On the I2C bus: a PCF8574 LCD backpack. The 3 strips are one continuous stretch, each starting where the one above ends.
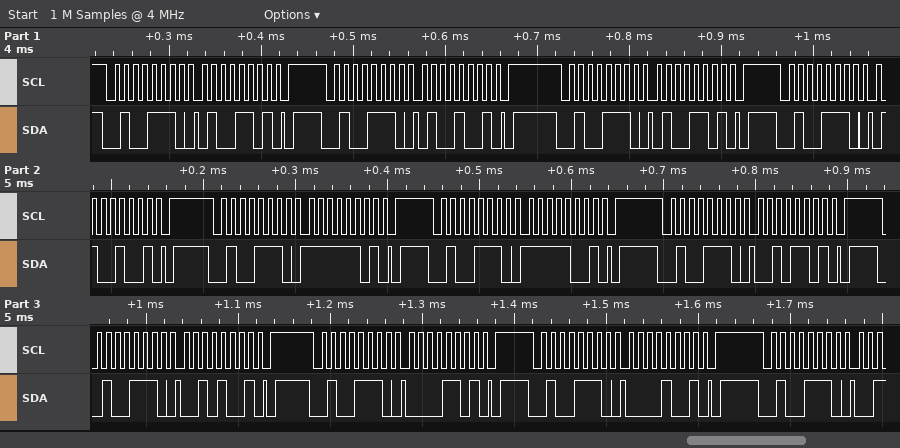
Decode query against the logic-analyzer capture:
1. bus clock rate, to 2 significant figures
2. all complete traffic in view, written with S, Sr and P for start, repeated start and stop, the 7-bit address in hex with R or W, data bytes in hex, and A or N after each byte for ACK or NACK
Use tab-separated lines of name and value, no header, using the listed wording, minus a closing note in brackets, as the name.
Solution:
bus clock rate, to 2 significant figures	100 kHz
all complete traffic in view, written with S, Sr and P for start, repeated start and stop, the 7-bit address in hex with R or W, data bytes in hex, and A or N after each byte for ACK or NACK	S 27W A 4D A P S 27W A 49 A P S 27W A 4D A P S 27W A 49 A P S 27W A FD A P S 27W A F9 A P S 27W A 2D A P S 27W A 29 A P S 27W A 0D A P S 27W A 09 A P S 27W A
